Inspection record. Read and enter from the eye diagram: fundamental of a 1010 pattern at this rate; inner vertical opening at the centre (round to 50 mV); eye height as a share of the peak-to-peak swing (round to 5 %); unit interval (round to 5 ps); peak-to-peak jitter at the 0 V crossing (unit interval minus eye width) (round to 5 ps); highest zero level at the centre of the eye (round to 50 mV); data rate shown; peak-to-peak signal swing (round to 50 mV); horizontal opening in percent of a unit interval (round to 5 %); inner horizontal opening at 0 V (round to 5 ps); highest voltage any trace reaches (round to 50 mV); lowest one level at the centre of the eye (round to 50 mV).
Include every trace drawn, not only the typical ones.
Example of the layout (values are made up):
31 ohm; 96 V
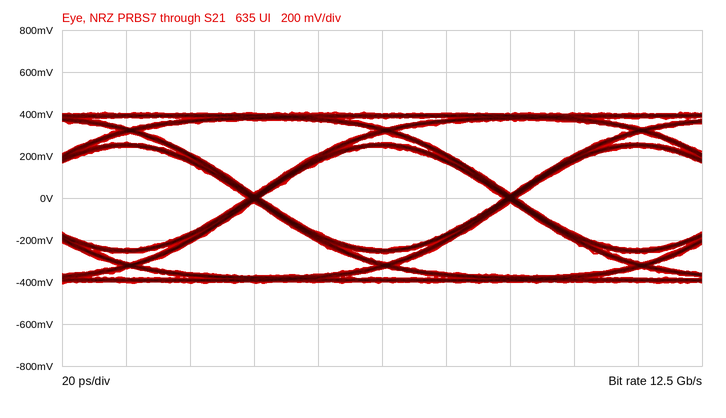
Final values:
6.25 GHz; 500 mV; 60 %; 80 ps; 5 ps; -250 mV; 12.5 Gb/s; 800 mV; 95 %; 75 ps; 400 mV; 250 mV
